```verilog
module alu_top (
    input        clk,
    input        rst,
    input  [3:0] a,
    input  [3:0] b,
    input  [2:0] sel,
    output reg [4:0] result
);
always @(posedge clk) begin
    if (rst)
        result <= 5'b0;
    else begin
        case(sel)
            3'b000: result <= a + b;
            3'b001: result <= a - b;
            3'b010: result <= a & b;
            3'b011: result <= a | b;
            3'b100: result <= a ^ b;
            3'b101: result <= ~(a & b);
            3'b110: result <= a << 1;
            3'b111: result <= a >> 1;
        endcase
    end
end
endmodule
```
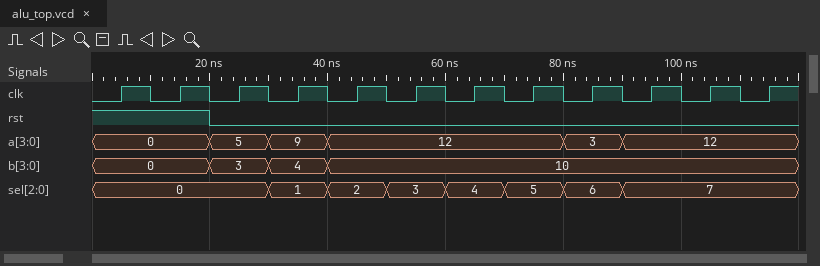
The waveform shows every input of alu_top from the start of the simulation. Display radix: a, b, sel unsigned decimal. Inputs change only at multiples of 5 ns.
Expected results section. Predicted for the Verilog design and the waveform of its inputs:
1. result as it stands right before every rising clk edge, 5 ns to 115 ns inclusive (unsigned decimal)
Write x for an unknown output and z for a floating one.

x, 0, 0, 8, 5, 8, 14, 6, 23, 6, 6, 6
